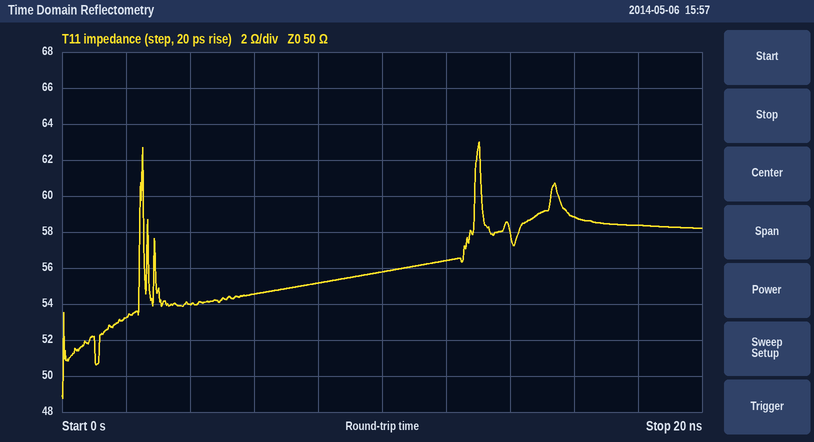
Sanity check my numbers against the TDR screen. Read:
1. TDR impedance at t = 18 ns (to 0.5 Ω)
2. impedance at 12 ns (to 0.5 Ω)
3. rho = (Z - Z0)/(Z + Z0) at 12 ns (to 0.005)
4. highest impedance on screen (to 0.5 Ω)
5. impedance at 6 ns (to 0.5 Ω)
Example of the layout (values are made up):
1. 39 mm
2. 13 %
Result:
1. 58.5 Ω
2. 56.5 Ω
3. +0.060
4. 63.0 Ω
5. 54.5 Ω
